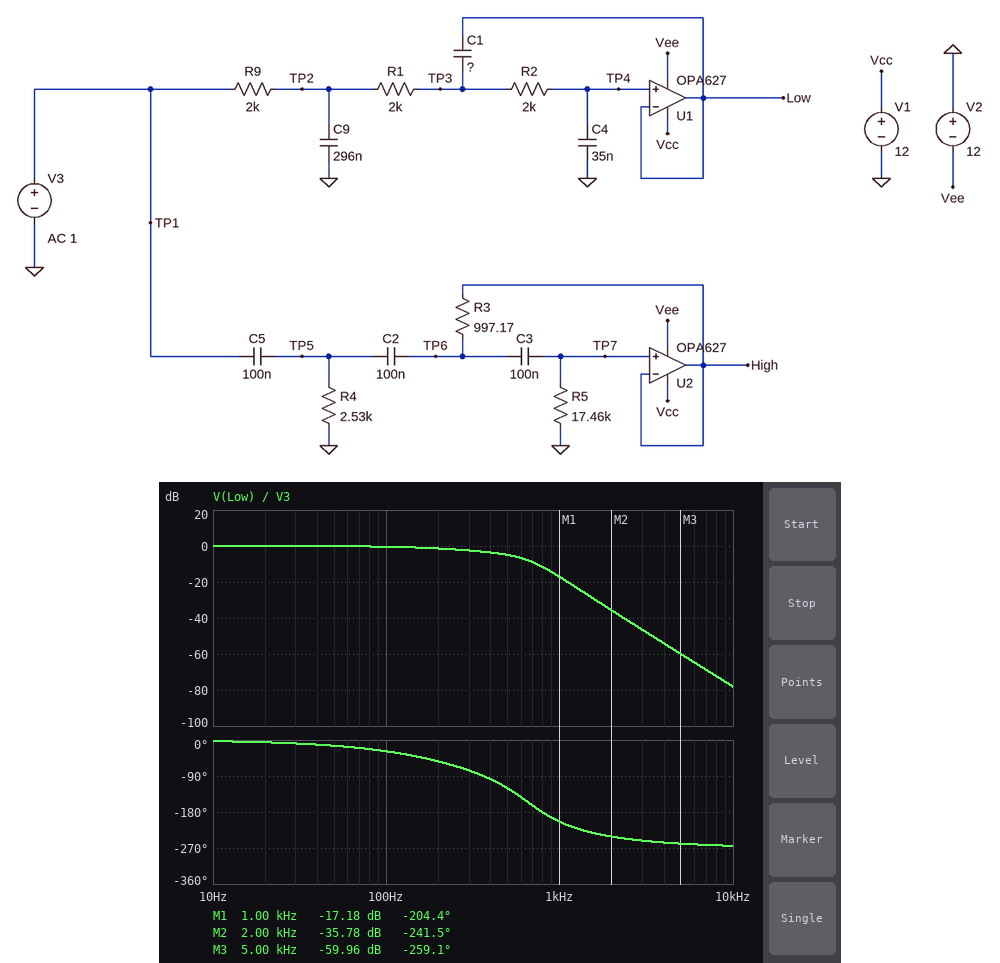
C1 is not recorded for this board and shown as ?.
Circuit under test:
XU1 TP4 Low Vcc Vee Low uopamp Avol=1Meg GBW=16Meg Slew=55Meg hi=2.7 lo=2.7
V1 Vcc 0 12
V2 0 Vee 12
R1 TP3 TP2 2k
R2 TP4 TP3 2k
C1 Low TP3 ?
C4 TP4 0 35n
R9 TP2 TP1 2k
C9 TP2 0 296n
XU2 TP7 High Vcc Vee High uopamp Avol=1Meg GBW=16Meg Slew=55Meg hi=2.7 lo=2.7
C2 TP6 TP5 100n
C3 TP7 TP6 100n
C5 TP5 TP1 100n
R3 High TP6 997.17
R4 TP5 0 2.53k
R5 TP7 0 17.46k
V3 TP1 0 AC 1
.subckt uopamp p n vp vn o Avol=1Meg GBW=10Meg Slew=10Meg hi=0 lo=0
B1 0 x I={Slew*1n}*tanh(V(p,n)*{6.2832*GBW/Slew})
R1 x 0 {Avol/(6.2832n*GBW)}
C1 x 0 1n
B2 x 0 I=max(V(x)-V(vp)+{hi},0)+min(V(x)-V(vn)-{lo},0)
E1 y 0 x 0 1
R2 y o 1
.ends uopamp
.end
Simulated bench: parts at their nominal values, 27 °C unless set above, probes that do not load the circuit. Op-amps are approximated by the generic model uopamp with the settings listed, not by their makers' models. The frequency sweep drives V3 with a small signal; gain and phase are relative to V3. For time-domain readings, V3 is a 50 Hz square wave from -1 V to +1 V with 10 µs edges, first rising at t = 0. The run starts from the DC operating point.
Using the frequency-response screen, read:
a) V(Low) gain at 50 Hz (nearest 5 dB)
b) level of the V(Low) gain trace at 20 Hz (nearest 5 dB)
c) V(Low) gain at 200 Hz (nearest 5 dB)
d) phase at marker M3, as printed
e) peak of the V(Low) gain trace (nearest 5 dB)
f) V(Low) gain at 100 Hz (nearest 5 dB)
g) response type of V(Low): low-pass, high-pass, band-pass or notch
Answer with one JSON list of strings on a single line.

["0 dB", "0 dB", "0 dB", "-259.1 deg", "0 dB", "0 dB", "low-pass"]
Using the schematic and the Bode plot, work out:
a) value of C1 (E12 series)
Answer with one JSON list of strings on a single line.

["390 nF"]
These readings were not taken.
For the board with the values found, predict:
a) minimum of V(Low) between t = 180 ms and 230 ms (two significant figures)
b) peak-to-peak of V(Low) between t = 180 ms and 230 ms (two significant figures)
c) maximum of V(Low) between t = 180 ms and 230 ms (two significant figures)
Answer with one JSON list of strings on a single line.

["-1.0 V", "2.0 V", "1.0 V"]
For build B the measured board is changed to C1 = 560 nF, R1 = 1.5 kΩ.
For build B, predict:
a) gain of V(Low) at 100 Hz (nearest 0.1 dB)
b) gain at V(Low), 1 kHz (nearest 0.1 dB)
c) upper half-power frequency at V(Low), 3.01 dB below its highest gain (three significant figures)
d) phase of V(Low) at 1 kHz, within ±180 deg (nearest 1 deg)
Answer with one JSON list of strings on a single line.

["-0.3 dB", "-18.2 dB", "381 Hz", "153 deg"]
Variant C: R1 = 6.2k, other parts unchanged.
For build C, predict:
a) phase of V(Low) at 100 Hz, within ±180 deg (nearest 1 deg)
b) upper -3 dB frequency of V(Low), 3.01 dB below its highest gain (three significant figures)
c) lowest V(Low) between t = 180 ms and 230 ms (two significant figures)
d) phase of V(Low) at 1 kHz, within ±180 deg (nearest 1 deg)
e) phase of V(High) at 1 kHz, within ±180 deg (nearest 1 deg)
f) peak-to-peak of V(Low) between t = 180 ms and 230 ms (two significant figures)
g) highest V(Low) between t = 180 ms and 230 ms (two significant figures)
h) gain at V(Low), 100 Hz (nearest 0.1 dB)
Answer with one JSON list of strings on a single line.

["-34 deg", "360 Hz", "-1.1 V", "128 deg", "54 deg", "2.2 V", "1.1 V", "-0.2 dB"]
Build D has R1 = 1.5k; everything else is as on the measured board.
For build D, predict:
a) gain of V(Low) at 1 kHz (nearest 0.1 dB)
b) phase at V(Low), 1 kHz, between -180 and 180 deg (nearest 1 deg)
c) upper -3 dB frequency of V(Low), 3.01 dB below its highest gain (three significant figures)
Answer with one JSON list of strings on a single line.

["-15.2 dB", "169 deg", "319 Hz"]
